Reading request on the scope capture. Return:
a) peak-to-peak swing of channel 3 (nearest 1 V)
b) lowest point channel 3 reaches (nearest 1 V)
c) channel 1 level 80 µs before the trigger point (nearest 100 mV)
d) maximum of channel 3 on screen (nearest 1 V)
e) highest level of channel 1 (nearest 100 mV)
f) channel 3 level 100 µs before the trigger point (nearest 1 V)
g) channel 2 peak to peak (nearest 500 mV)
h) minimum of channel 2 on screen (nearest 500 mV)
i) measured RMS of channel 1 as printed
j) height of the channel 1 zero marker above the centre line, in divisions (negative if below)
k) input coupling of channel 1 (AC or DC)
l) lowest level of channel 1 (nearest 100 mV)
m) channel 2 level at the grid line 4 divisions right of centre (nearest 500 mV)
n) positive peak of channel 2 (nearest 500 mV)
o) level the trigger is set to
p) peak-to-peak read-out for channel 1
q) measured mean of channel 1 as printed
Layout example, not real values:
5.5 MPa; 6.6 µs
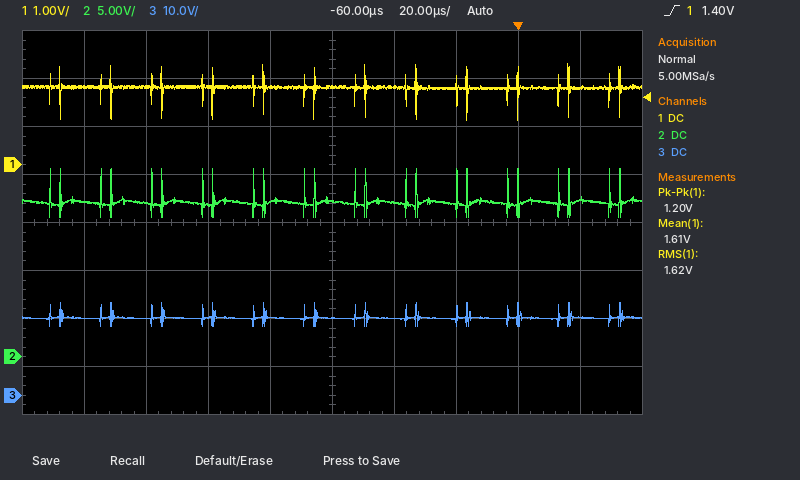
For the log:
5 V; 14 V; 1.6 V; 19 V; 2.1 V; 16 V; 5.0 V; 14.5 V; 1.62 V; +1.2 div; DC; 900 mV; 16.5 V; 19.5 V; 1.40 V; 1.20 V; 1.61 V
